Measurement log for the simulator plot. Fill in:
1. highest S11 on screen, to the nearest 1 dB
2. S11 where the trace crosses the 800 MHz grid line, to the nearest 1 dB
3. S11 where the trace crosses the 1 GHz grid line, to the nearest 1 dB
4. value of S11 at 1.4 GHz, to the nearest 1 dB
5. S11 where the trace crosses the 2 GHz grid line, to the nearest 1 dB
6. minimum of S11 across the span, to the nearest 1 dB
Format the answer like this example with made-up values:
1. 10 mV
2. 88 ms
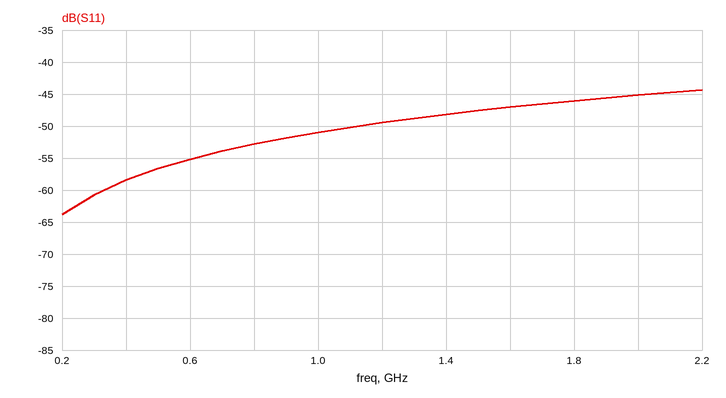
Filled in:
1. -44 dB
2. -53 dB
3. -51 dB
4. -48 dB
5. -45 dB
6. -64 dB
